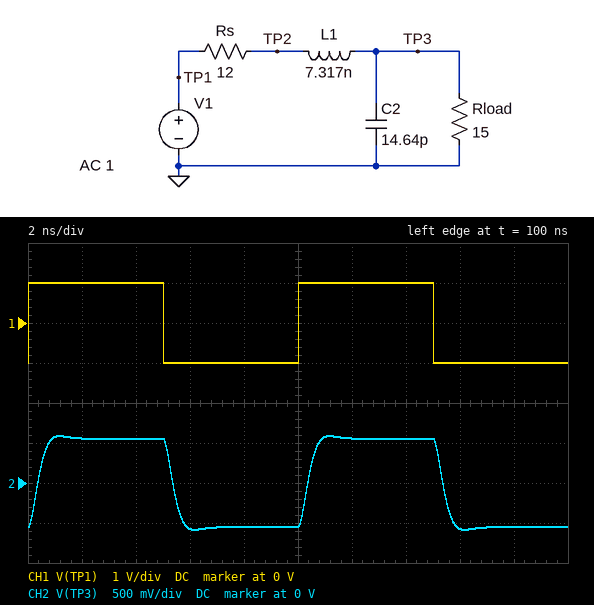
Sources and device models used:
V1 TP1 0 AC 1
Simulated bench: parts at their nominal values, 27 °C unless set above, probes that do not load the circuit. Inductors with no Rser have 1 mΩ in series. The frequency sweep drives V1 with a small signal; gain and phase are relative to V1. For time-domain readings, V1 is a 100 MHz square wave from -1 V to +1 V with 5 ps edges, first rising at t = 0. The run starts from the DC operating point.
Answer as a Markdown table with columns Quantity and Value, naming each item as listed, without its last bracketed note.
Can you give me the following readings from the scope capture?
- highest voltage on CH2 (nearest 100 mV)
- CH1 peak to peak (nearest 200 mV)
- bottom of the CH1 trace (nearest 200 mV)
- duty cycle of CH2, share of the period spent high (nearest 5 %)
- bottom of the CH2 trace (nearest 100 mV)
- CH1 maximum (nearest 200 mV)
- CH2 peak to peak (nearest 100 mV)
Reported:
| Quantity | Value |
|---|---|
| highest voltage on CH2 | 600 mV |
| CH1 peak to peak | 2.0 V |
| bottom of the CH1 trace | -1.0 V |
| duty cycle of CH2, share of the period spent high | 50 % |
| bottom of the CH2 trace | -600 mV |
| CH1 maximum | 1.0 V |
| CH2 peak to peak | 1.2 V |
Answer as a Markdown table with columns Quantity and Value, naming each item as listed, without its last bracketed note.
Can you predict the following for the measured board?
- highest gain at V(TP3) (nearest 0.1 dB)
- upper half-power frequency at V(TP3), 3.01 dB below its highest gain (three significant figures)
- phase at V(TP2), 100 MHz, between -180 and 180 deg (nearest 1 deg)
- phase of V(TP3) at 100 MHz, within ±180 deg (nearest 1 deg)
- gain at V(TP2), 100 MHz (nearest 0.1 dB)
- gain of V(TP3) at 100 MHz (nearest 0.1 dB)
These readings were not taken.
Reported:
| Quantity | Value |
|---|---|
| highest gain at V(TP3) | -5.1 dB |
| upper half-power frequency at V(TP3), 3.01 dB below its highest gain | 608 MHz |
| phase at V(TP2), 100 MHz, between -180 and 180 deg | 4 deg |
| phase of V(TP3) at 100 MHz, within ±180 deg | -13 deg |
| gain at V(TP2), 100 MHz | -5.1 dB |
| gain of V(TP3) at 100 MHz | -5.1 dB |
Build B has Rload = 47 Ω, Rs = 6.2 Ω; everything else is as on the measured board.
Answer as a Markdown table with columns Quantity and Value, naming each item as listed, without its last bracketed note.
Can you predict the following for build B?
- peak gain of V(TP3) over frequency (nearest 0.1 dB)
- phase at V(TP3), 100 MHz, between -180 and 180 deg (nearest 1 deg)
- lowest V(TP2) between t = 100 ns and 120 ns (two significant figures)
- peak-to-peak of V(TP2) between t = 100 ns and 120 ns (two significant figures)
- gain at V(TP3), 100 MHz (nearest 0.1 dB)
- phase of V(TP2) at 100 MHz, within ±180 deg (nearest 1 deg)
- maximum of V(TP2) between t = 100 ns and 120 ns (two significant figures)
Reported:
| Quantity | Value |
|---|---|
| peak gain of V(TP3) over frequency | 2.5 dB |
| phase at V(TP3), 100 MHz, between -180 and 180 deg | -8 deg |
| lowest V(TP2) between t = 100 ns and 120 ns | -1.1 V |
| peak-to-peak of V(TP2) between t = 100 ns and 120 ns | 2.2 V |
| gain at V(TP3), 100 MHz | -0.8 dB |
| phase of V(TP2) at 100 MHz, within ±180 deg | -2 deg |
| maximum of V(TP2) between t = 100 ns and 120 ns | 1.1 V |
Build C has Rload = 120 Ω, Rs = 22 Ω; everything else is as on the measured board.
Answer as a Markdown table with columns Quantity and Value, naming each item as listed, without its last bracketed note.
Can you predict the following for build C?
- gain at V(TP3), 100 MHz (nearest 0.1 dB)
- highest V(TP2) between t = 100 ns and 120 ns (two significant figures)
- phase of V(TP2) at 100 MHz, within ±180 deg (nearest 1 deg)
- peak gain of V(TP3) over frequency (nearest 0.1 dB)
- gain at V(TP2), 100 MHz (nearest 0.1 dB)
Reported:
| Quantity | Value |
|---|---|
| gain at V(TP3), 100 MHz | -1.3 dB |
| highest V(TP2) between t = 100 ns and 120 ns | 1.1 V |
| phase of V(TP2) at 100 MHz, within ±180 deg | -10 deg |
| peak gain of V(TP3) over frequency | -0.6 dB |
| gain at V(TP2), 100 MHz | -1.7 dB |
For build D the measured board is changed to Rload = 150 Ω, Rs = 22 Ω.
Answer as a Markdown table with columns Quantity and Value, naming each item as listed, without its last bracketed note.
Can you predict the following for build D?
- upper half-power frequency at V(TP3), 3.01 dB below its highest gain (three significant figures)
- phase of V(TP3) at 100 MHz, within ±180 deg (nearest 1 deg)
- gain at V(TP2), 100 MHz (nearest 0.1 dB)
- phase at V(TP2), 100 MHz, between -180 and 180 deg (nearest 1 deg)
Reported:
| Quantity | Value |
|---|---|
| upper half-power frequency at V(TP3), 3.01 dB below its highest gain | 602 MHz |
| phase of V(TP3) at 100 MHz, within ±180 deg | -12 deg |
| gain at V(TP2), 100 MHz | -1.4 dB |
| phase at V(TP2), 100 MHz, between -180 and 180 deg | -10 deg |
